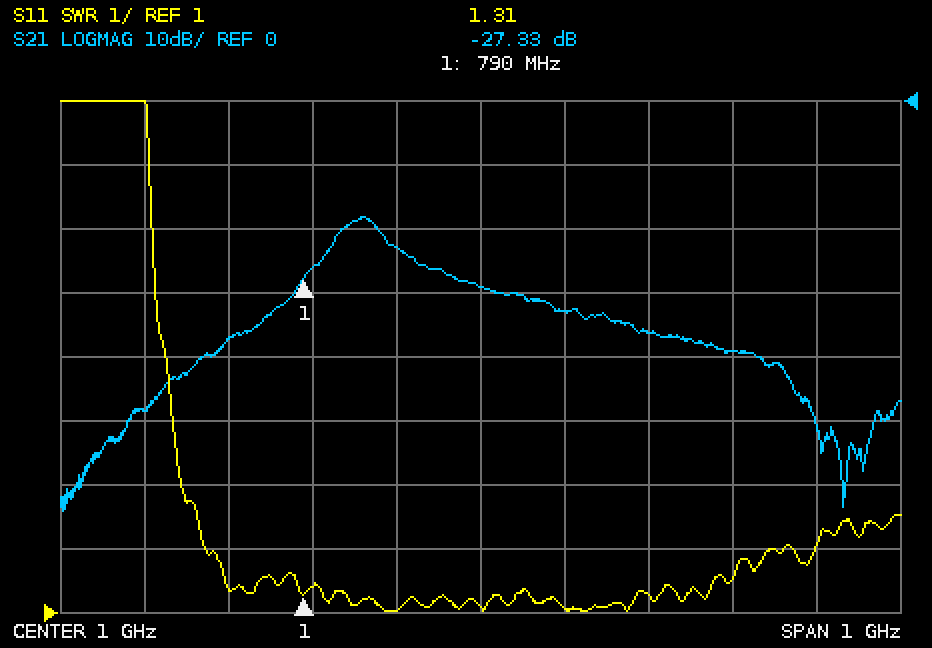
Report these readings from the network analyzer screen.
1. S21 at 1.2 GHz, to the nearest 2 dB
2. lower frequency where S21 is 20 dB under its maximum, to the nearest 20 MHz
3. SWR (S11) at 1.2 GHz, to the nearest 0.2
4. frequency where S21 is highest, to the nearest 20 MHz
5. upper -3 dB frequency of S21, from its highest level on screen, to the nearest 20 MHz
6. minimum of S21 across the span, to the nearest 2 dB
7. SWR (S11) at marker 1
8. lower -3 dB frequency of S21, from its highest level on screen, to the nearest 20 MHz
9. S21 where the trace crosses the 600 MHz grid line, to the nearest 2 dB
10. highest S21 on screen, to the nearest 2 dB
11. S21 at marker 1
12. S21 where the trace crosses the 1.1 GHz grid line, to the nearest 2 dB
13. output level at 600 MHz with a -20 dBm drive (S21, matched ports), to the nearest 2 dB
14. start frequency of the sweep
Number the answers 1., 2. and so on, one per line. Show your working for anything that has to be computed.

1. -36 dB
2. 700 MHz
3. 1.2
4. 860 MHz
5. 880 MHz
6. -64 dB
7. 1.31
8. 820 MHz
9. -48 dB
10. -18 dB
11. -27.33 dB
12. -32 dB
13. -20 dBm + (-48 dB) = -68 dBm
14. 500 MHz
